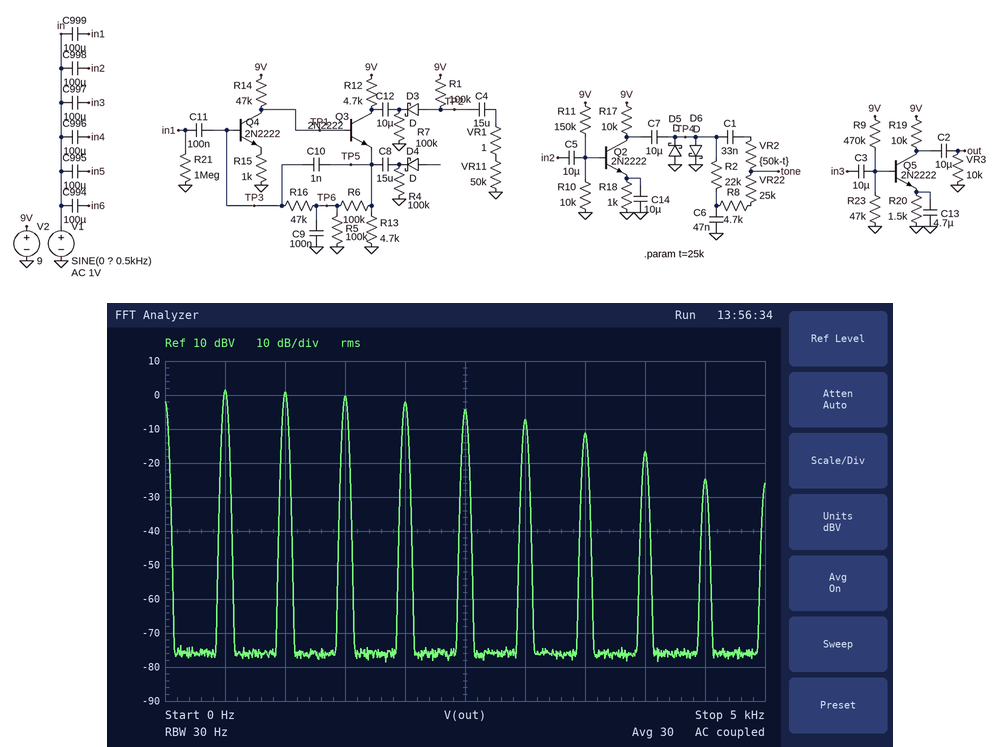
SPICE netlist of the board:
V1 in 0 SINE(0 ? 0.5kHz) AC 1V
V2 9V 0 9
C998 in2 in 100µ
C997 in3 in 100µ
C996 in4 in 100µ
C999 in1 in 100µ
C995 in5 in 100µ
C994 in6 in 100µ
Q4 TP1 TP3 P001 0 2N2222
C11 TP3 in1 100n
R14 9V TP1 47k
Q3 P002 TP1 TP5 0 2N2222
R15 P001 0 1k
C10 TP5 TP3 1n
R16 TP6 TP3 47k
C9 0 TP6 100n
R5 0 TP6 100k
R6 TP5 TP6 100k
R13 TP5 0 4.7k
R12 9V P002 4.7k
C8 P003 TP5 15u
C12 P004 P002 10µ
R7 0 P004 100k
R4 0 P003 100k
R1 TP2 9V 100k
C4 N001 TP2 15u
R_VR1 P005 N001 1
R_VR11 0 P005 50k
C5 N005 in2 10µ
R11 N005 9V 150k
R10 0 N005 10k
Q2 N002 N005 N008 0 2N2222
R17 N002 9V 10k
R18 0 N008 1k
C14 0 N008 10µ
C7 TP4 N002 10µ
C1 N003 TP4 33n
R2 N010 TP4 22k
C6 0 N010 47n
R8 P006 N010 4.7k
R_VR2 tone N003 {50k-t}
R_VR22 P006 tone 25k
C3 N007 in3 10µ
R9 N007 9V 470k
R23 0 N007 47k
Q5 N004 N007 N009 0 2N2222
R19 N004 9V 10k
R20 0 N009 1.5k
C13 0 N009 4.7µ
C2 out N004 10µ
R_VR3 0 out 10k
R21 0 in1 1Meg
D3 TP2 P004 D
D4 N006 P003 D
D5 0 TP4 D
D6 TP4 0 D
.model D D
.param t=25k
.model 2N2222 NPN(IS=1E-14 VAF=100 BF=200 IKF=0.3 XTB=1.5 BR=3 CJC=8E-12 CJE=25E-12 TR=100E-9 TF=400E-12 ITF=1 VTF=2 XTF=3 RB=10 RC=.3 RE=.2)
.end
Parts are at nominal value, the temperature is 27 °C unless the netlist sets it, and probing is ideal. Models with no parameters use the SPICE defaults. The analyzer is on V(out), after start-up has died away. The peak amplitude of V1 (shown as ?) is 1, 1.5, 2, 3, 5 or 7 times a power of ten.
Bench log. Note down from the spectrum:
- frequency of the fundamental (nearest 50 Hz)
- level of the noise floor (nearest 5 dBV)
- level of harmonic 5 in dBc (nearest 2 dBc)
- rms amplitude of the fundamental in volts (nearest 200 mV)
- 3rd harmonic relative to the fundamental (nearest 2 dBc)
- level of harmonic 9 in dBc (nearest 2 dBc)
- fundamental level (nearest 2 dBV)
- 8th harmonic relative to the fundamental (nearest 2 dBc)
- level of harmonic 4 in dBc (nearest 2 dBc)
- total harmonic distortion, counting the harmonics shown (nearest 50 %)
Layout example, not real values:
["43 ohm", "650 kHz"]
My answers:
["500 Hz", "-75 dBV", "-6 dBc", "1.2 V", "-2 dBc", "-26 dBc", "2 dBV", "-18 dBc", "-4 dBc", "150 %"]
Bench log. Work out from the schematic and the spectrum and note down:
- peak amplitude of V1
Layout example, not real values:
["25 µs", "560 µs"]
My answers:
["700 mV"]
